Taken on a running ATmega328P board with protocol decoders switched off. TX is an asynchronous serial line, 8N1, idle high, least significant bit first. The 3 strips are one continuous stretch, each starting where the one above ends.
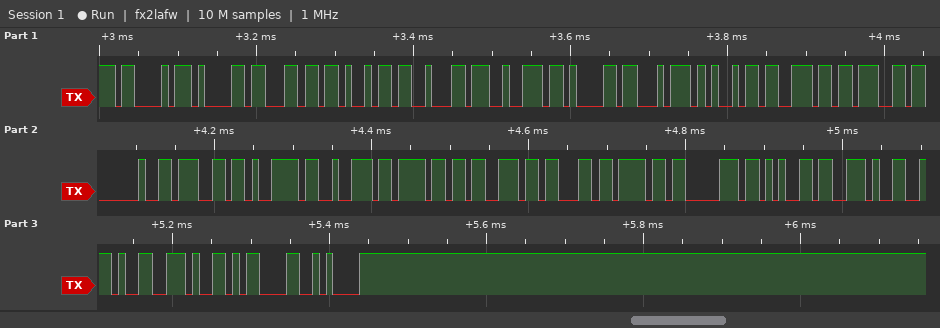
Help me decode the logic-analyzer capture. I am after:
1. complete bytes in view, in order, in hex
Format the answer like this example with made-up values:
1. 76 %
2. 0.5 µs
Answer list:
1. 43 61 6C 69 62 72 61 74 69 6E 67 20 67 79 72 6F 73 63 6F 70 65 2E 2E 2E 0D 0A
